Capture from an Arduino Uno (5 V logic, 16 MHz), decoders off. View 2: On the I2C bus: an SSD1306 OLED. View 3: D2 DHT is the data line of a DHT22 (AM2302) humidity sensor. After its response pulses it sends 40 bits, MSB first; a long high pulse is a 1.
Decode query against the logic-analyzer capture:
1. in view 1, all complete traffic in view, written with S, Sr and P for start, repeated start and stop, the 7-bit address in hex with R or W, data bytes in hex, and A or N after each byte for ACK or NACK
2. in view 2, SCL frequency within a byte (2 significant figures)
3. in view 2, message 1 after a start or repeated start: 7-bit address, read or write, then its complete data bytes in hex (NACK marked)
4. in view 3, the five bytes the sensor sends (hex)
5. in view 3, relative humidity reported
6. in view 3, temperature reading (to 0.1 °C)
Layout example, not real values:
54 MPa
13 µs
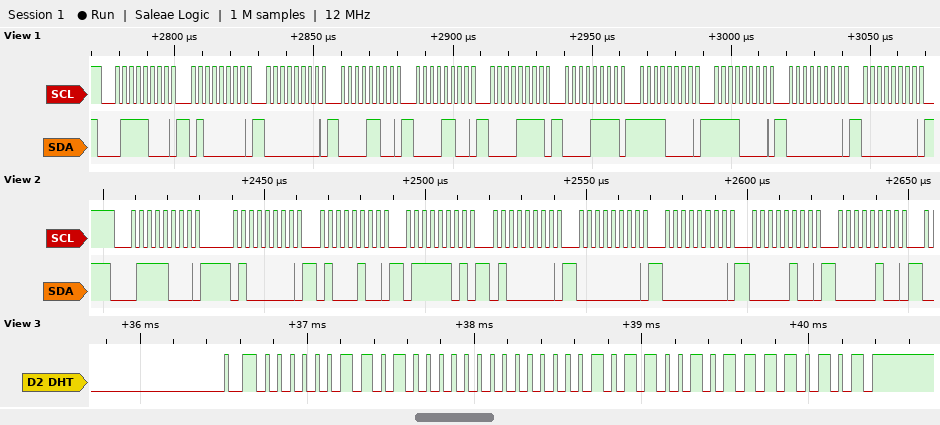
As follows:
S 3CW A 40 A 00 A 0C A 0C A 0F A 0F A F0 A F0 A 00 A 00 A
400 kHz
0x3C write: 40 44 7D 40 00 00 04 04
03 40 00 B2 F5
83.2 %
17.8 °C
